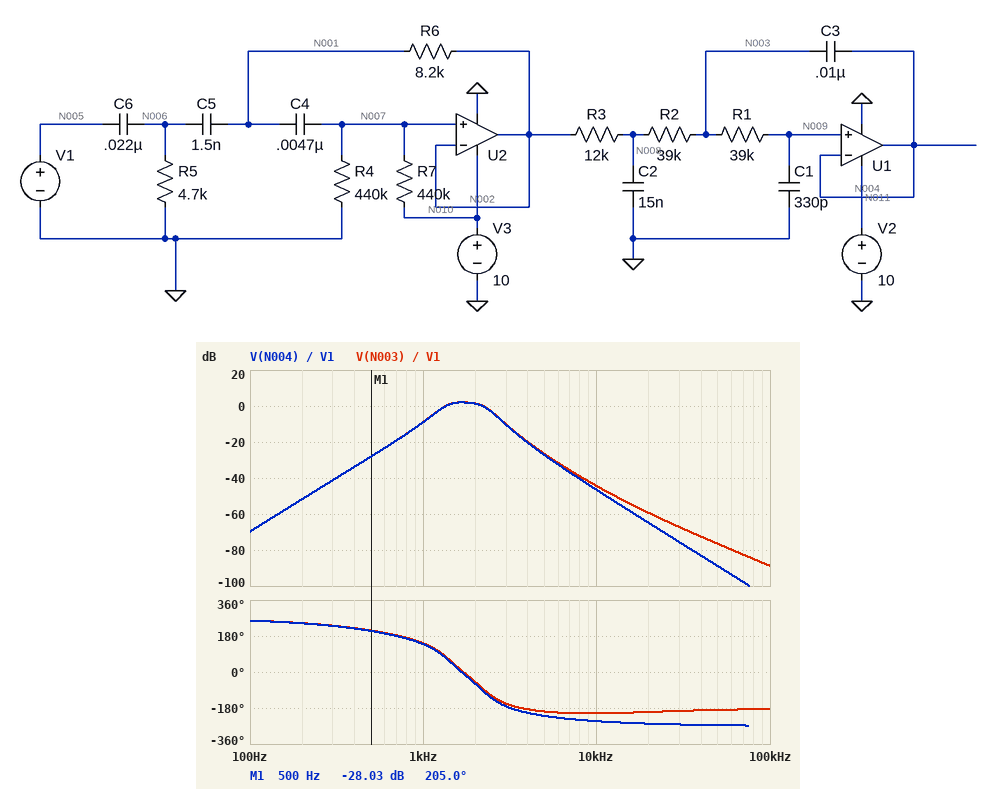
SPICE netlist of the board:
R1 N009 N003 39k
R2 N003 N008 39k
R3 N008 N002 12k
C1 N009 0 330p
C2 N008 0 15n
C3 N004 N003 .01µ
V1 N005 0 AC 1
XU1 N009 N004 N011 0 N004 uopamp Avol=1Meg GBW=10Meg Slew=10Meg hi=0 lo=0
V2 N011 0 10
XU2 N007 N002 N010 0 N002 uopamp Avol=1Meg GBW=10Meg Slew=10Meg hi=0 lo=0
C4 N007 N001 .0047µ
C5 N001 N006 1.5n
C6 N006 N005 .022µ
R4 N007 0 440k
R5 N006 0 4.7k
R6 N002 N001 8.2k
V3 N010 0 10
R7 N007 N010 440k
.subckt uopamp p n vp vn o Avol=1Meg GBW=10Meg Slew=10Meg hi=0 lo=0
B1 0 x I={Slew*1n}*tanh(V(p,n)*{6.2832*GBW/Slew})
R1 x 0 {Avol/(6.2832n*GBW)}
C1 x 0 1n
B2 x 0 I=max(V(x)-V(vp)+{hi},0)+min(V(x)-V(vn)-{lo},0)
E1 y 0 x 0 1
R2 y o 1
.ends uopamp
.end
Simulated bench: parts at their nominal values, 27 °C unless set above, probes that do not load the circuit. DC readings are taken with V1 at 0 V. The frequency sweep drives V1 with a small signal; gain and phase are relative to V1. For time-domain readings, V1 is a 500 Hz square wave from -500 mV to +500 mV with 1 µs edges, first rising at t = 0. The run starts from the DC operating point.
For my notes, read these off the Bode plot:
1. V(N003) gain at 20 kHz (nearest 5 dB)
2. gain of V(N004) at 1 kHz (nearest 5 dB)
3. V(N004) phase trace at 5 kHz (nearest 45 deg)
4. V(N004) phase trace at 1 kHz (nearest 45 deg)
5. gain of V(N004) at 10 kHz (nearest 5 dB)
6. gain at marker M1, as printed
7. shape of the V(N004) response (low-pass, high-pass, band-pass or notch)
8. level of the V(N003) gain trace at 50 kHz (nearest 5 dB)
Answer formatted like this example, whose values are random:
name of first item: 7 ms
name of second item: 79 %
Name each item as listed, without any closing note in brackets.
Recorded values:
V(N003) gain at 20 kHz: -60 dB
gain of V(N004) at 1 kHz: -10 dB
V(N004) phase trace at 5 kHz: -225 deg
V(N004) phase trace at 1 kHz: 135 deg
gain of V(N004) at 10 kHz: -45 dB
gain at marker M1, as printed: -28.03 dB
shape of the V(N004) response: band-pass
level of the V(N003) gain trace at 50 kHz: -75 dB
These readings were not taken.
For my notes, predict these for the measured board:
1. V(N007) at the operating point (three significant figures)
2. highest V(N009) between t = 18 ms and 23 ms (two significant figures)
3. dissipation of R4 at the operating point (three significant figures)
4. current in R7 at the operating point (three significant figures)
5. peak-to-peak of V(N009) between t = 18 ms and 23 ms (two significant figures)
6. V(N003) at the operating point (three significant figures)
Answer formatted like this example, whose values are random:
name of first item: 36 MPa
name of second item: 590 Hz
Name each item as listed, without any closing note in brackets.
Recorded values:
V(N007) at the operating point: 5.00 V
highest V(N009) between t = 18 ms and 23 ms: 5.4 V
dissipation of R4 at the operating point: 56.8 µW
current in R7 at the operating point: 11.4 µA
peak-to-peak of V(N009) between t = 18 ms and 23 ms: 720 mV
V(N003) at the operating point: 5.00 V
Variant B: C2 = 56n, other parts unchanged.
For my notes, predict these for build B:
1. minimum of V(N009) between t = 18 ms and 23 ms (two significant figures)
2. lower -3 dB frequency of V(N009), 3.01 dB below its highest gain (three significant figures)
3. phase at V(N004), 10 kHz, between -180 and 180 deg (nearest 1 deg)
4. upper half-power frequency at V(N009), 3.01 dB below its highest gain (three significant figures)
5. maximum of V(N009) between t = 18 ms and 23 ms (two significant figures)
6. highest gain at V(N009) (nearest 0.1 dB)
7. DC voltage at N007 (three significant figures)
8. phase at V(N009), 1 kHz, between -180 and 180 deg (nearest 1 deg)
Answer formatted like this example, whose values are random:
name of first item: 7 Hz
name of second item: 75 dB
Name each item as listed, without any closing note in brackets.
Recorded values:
minimum of V(N009) between t = 18 ms and 23 ms: 4.9 V
lower -3 dB frequency of V(N009), 3.01 dB below its highest gain: 1.28 kHz
phase at V(N004), 10 kHz, between -180 and 180 deg: 109 deg
upper half-power frequency at V(N009), 3.01 dB below its highest gain: 2.37 kHz
maximum of V(N009) between t = 18 ms and 23 ms: 5.1 V
highest gain at V(N009): -8.2 dB
DC voltage at N007: 5.00 V
phase at V(N009), 1 kHz, between -180 and 180 deg: 113 deg
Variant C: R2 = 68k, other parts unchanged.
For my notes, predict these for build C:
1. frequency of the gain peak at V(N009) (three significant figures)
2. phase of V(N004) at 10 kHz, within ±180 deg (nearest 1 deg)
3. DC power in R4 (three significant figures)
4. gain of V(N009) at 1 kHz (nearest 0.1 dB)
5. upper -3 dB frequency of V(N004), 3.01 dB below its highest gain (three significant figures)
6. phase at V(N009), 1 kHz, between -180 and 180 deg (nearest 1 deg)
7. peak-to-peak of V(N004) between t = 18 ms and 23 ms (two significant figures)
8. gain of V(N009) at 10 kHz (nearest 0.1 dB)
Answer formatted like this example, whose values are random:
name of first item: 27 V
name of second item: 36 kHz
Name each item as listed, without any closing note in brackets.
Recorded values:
frequency of the gain peak at V(N009): 1.54 kHz
phase of V(N004) at 10 kHz, within ±180 deg: 112 deg
DC power in R4: 56.8 µW
gain of V(N009) at 1 kHz: -7.5 dB
upper -3 dB frequency of V(N004), 3.01 dB below its highest gain: 1.82 kHz
phase at V(N009), 1 kHz, between -180 and 180 deg: 131 deg
peak-to-peak of V(N004) between t = 18 ms and 23 ms: 810 mV
gain of V(N009) at 10 kHz: -51.6 dB
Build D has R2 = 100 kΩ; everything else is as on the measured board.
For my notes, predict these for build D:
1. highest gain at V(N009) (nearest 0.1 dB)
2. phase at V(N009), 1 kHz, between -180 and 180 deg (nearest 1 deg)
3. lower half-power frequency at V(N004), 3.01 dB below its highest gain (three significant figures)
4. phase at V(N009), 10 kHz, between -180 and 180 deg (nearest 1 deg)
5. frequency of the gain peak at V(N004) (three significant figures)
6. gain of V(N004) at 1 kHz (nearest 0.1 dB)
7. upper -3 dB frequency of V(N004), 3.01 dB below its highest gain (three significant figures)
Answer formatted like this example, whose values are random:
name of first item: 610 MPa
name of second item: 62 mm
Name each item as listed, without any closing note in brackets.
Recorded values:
highest gain at V(N009): 3.7 dB
phase at V(N009), 1 kHz, between -180 and 180 deg: 119 deg
lower half-power frequency at V(N004), 3.01 dB below its highest gain: 1.20 kHz
phase at V(N009), 10 kHz, between -180 and 180 deg: 112 deg
frequency of the gain peak at V(N004): 1.40 kHz
gain of V(N004) at 1 kHz: -6.0 dB
upper -3 dB frequency of V(N004), 3.01 dB below its highest gain: 1.63 kHz
